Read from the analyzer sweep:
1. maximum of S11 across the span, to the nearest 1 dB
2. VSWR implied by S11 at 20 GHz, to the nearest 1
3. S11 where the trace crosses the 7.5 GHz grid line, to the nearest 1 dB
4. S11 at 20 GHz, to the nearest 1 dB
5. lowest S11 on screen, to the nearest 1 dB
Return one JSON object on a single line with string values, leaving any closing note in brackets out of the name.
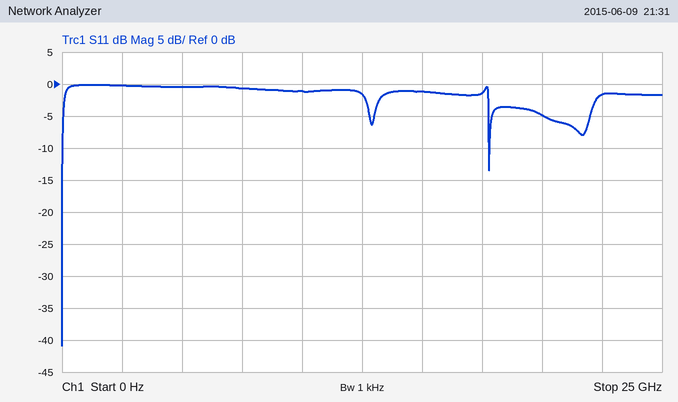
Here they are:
{"maximum of S11 across the span, to the nearest 1 dB": "0 dB", "VSWR implied by S11 at 20 GHz, to the nearest 1": "4", "S11 where the trace crosses the 7.5 GHz grid line, to the nearest 1 dB": "-1 dB", "S11 at 20 GHz, to the nearest 1 dB": "-5 dB", "lowest S11 on screen, to the nearest 1 dB": "-41 dB"}
